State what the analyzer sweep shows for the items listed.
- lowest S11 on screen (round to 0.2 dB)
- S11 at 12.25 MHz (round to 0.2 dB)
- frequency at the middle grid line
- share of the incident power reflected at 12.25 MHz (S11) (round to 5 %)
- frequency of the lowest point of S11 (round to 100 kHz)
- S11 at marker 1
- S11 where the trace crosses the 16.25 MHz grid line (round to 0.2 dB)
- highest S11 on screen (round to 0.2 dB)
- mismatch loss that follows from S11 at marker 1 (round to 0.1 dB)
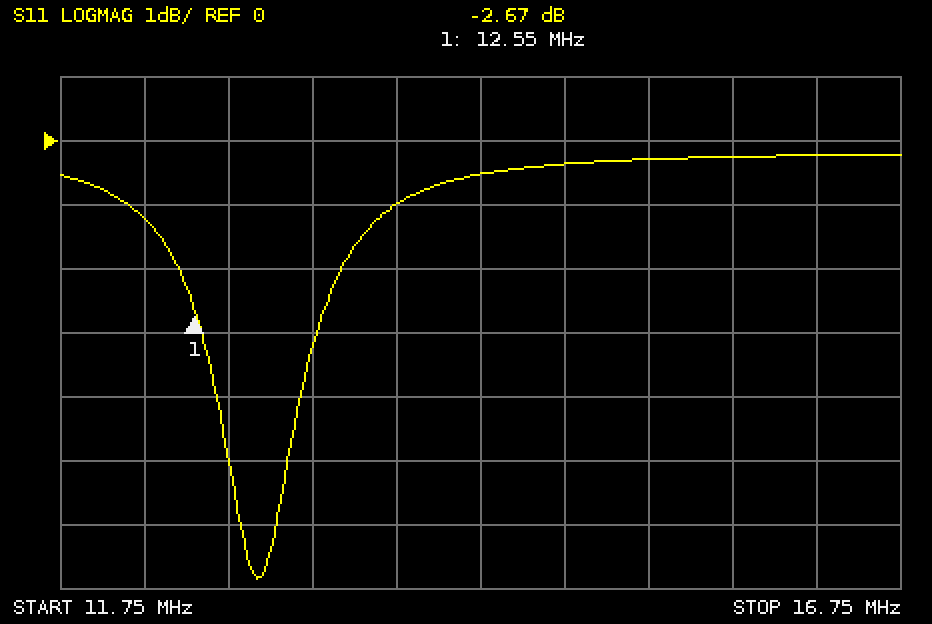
-6.8 dB
-1.2 dB
14.25 MHz
75 %
12.9 MHz
-2.67 dB
-0.2 dB
-0.2 dB
3.4 dB
